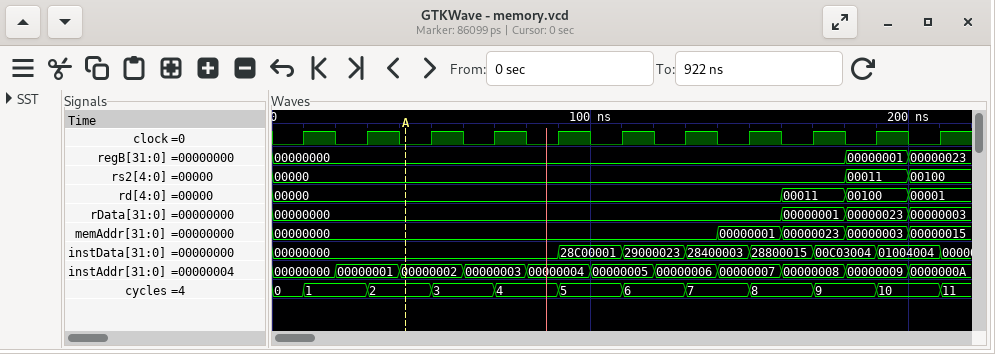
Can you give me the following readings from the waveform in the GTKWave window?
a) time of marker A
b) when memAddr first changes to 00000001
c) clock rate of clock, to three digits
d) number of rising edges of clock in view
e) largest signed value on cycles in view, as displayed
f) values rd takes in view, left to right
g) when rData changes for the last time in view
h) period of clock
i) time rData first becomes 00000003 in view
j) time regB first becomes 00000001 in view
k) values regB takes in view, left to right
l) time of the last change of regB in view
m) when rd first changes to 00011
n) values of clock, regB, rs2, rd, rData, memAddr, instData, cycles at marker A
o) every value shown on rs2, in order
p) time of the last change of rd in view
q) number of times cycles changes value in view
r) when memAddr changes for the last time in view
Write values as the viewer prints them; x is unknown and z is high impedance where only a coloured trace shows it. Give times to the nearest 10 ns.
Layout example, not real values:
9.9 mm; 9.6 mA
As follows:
40 ns; 140 ns; 50.0 MHz; 11; 11; 00000, 00011, 00100, 00001; 200 ns; 20 ns; 200 ns; 180 ns; 00000000, 00000001, 00000023; 200 ns; 160 ns; clock=0, regB=00000000, rs2=00000, rd=00000, rData=00000000, memAddr=00000000, instData=00000000, cycles=2; 00000, 00011, 00100; 200 ns; 11; 200 ns
